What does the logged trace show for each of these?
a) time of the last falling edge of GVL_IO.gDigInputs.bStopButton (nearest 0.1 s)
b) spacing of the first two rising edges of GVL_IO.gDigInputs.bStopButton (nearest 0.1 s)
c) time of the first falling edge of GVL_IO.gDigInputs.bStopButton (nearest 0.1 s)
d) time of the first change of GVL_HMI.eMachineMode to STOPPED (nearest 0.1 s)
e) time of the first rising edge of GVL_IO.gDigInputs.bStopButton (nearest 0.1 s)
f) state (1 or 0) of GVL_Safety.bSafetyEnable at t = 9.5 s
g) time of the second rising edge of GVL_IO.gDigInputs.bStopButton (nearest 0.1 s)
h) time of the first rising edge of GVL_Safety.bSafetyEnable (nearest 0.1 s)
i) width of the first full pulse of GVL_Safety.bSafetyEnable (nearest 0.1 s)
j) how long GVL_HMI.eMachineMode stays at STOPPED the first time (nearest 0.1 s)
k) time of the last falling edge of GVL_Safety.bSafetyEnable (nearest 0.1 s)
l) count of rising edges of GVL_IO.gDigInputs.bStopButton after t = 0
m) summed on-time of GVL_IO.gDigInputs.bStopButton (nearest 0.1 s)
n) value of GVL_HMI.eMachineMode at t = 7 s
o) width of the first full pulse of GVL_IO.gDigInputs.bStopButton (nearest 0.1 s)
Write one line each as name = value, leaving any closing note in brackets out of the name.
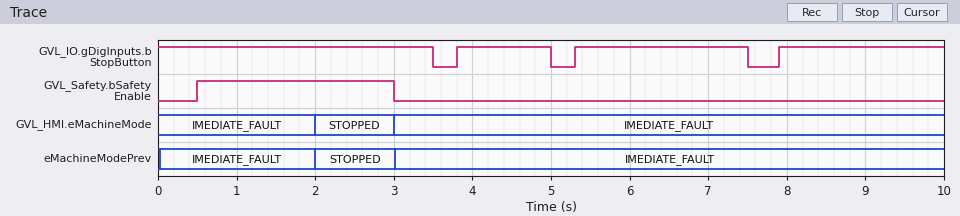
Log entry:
time of the last falling edge of GVL_IO.gDigInputs.bStopButton = 7.5 s
spacing of the first two rising edges of GVL_IO.gDigInputs.bStopButton = 1.5 s
time of the first falling edge of GVL_IO.gDigInputs.bStopButton = 3.5 s
time of the first change of GVL_HMI.eMachineMode to STOPPED = 2.0 s
time of the first rising edge of GVL_IO.gDigInputs.bStopButton = 3.8 s
state (1 or 0) of GVL_Safety.bSafetyEnable at t = 9.5 s = 0
time of the second rising edge of GVL_IO.gDigInputs.bStopButton = 5.3 s
time of the first rising edge of GVL_Safety.bSafetyEnable = 0.5 s
width of the first full pulse of GVL_Safety.bSafetyEnable = 2.5 s
how long GVL_HMI.eMachineMode stays at STOPPED the first time = 1.0 s
time of the last falling edge of GVL_Safety.bSafetyEnable = 3.0 s
count of rising edges of GVL_IO.gDigInputs.bStopButton after t = 0 = 3
summed on-time of GVL_IO.gDigInputs.bStopButton = 9.0 s
value of GVL_HMI.eMachineMode at t = 7 s = IMEDIATE_FAULT
width of the first full pulse of GVL_IO.gDigInputs.bStopButton = 1.2 s
